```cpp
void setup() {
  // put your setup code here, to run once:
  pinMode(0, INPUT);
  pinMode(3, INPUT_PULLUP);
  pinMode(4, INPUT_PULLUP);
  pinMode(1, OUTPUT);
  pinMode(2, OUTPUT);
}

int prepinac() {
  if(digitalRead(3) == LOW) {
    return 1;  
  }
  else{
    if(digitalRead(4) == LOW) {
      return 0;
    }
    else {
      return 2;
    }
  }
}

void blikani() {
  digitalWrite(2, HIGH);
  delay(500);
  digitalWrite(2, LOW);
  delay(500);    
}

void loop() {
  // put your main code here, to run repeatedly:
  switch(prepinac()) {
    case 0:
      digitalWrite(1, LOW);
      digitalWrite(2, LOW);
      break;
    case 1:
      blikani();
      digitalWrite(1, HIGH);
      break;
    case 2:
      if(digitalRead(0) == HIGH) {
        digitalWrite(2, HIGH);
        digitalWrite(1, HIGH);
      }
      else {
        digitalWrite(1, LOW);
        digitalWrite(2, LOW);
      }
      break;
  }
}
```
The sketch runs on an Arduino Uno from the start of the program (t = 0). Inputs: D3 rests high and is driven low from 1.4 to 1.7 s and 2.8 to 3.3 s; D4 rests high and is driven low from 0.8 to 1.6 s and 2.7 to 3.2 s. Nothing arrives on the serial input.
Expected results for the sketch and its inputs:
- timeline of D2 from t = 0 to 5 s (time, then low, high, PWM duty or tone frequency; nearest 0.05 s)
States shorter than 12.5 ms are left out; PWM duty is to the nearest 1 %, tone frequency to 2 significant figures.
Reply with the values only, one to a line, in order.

0 s low; 1.4 s high; 1.9 s low; 2.8 s high; 3.3 s low
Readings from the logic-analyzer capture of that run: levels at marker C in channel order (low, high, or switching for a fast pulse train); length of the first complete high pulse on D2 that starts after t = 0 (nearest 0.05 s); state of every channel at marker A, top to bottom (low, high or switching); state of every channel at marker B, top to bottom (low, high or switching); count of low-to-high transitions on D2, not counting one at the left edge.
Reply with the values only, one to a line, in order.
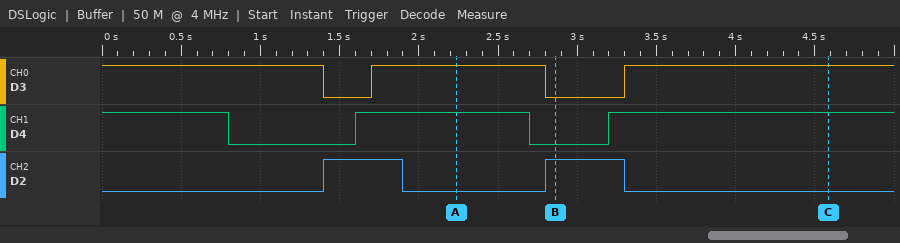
D3 high, D4 high, D2 low
0.50 s
D3 high, D4 high, D2 low
D3 low, D4 low, D2 high
2
